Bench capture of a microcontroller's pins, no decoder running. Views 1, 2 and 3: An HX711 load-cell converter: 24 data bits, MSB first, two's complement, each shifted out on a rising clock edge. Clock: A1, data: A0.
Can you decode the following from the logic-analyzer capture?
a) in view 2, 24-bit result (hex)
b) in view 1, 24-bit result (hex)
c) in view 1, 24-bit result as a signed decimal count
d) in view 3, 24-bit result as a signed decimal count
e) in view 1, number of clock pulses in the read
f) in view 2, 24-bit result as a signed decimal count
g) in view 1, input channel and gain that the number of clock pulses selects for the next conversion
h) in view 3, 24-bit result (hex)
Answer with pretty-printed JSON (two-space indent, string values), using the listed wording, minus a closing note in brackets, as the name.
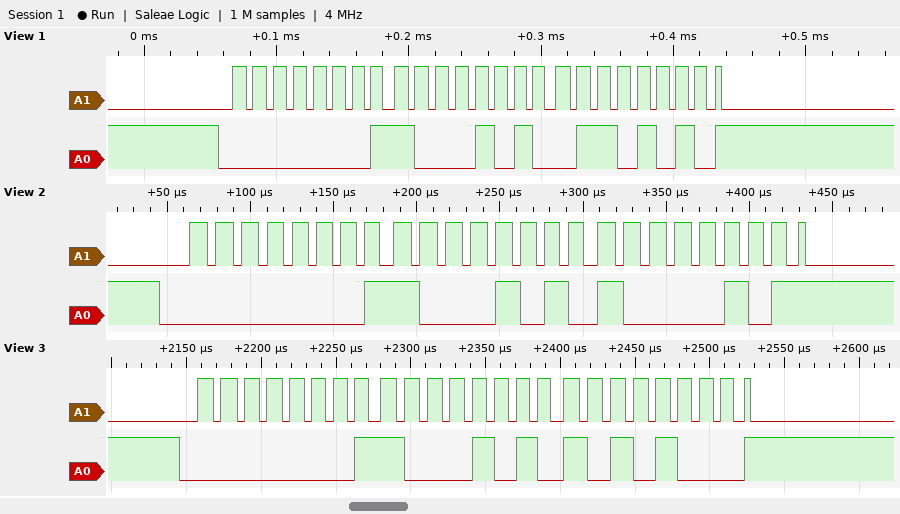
{
  "in view 2, 24-bit result": "0x018A85",
  "in view 1, 24-bit result": "0x018A6A",
  "in view 1, 24-bit result as a signed decimal count": "100970",
  "in view 3, 24-bit result as a signed decimal count": "101032",
  "in view 1, number of clock pulses in the read": "25",
  "in view 2, 24-bit result as a signed decimal count": "100997",
  "in view 1, input channel and gain that the number of clock pulses selects for the next conversion": "channel A, gain 128",
  "in view 3, 24-bit result": "0x018AA8"
}
